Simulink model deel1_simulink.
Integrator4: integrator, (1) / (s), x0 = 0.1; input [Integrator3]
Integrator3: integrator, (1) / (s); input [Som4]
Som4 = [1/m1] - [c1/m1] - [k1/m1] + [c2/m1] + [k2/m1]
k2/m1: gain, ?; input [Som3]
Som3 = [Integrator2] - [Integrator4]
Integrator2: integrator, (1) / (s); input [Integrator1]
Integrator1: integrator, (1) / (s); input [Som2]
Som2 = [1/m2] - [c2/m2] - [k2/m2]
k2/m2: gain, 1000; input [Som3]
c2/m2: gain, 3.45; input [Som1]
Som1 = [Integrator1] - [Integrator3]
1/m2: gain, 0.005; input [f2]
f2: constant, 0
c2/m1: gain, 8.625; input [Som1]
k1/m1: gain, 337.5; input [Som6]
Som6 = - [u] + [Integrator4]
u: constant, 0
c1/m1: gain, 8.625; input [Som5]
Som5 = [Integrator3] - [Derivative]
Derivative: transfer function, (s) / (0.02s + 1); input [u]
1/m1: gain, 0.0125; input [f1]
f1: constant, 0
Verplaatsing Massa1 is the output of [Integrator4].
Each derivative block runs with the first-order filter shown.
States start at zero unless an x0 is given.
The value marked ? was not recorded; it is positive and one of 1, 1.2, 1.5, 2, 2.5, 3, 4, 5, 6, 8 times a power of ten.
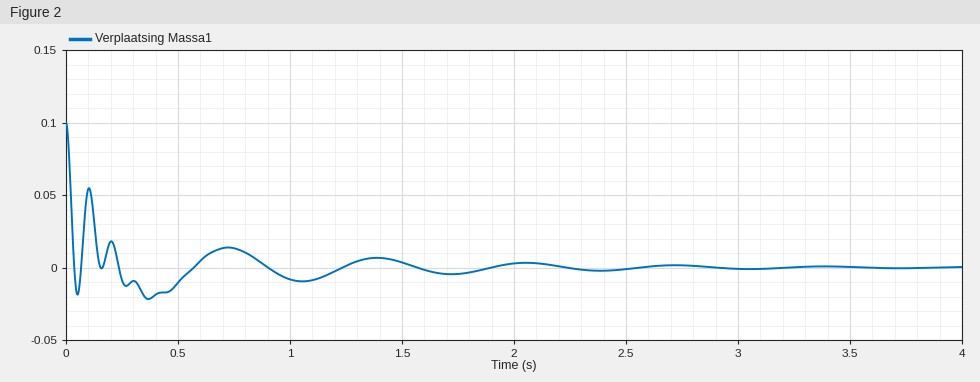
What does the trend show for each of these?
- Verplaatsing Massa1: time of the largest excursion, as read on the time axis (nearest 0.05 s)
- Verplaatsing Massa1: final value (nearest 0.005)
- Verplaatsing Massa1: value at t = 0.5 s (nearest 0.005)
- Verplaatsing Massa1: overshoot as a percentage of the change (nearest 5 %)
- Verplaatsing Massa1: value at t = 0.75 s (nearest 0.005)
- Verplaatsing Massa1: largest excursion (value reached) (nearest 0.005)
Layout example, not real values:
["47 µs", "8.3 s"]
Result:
["0.35 s", "0.000", "-0.010", "20 %", "0.015", "-0.020"]
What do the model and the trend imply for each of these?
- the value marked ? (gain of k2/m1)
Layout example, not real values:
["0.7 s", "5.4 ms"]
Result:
["2500"]
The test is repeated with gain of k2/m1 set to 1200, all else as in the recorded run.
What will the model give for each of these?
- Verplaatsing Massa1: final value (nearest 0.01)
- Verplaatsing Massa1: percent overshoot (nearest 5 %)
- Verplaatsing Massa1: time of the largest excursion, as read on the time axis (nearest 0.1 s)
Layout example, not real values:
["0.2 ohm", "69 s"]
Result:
["0.00", "35 %", "0.3 s"]
